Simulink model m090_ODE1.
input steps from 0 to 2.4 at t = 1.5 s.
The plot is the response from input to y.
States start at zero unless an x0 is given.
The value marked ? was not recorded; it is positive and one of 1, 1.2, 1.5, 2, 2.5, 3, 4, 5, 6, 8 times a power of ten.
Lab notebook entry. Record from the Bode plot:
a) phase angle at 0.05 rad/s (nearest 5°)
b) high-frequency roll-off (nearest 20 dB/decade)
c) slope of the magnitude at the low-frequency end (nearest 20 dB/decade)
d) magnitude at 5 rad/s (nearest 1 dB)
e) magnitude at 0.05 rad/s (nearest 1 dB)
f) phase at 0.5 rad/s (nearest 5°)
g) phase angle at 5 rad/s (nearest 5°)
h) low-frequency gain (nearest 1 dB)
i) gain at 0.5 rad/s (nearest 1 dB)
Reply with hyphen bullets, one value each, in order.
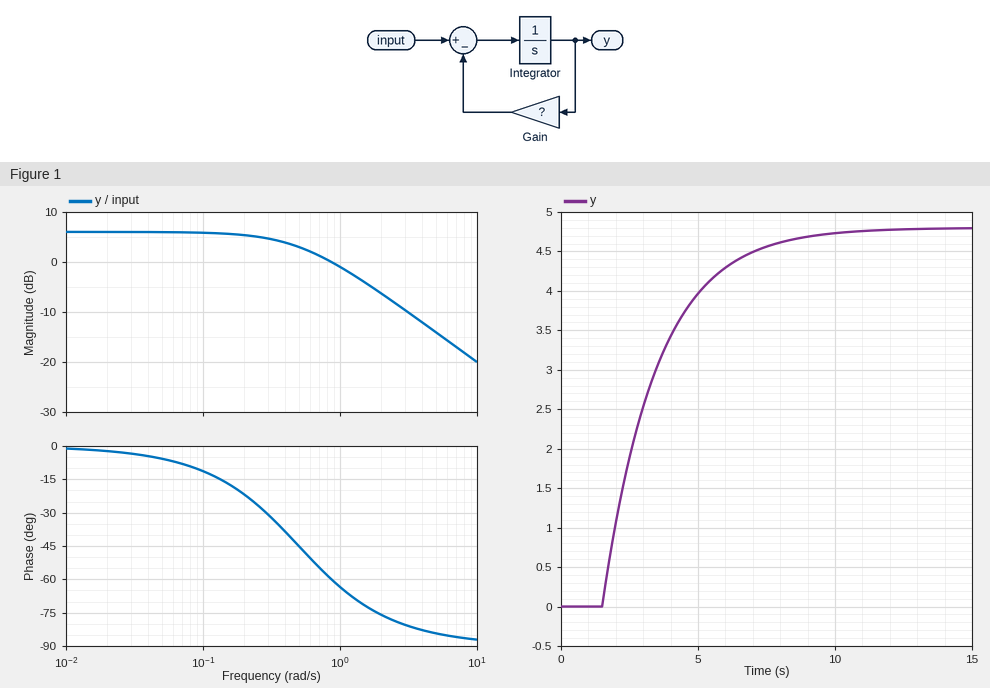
- -5°
- -20 dB/decade
- 0 dB/decade
- -14 dB
- 6 dB
- -45°
- -85°
- 6 dB
- 3 dB
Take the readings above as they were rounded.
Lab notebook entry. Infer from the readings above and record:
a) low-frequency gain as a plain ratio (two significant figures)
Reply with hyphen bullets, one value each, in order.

- 2.0
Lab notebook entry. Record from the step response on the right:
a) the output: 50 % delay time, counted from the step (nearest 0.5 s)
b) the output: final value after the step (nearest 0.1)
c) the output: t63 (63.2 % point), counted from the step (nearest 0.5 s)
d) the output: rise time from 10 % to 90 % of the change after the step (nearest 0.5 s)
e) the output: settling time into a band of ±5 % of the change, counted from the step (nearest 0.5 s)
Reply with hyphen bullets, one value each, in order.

- 1.5 s
- 4.8
- 2.0 s
- 4.5 s
- 6.0 s
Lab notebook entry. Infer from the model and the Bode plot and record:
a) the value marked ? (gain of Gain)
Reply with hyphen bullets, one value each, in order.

- 0.5
